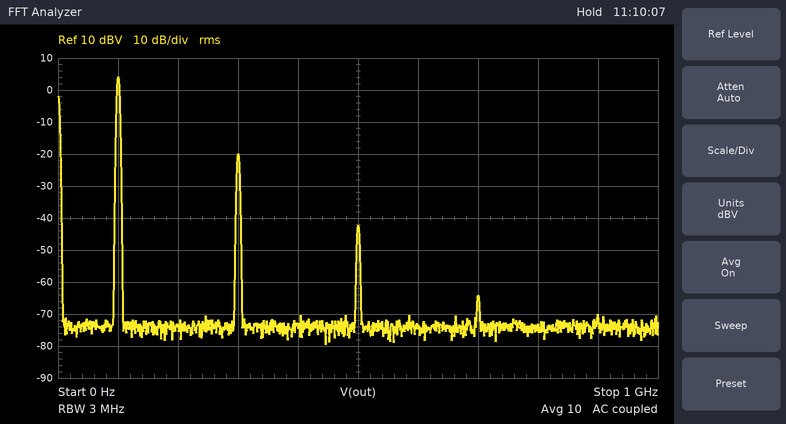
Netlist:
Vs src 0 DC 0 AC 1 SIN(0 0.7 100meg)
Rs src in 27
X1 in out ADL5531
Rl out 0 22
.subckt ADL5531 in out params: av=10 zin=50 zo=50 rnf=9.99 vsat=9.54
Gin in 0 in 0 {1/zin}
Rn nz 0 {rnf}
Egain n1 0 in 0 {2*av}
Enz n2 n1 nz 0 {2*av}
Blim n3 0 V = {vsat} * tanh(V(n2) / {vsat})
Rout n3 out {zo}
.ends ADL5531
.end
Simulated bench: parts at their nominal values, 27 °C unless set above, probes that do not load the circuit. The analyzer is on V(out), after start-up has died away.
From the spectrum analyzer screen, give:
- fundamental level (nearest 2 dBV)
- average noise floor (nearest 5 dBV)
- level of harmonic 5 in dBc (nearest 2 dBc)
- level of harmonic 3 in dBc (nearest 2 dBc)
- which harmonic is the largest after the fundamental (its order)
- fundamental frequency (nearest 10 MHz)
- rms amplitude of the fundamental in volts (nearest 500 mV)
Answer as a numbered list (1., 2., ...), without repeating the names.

1. 4 dBV
2. -75 dBV
3. -46 dBc
4. -24 dBc
5. 3
6. 100 MHz
7. 1.5 V
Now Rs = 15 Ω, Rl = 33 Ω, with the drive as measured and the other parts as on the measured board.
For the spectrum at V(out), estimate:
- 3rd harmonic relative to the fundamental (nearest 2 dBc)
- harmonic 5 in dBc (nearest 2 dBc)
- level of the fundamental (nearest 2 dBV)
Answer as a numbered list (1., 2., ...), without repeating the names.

1. -22 dBc
2. -42 dBc
3. 8 dBV
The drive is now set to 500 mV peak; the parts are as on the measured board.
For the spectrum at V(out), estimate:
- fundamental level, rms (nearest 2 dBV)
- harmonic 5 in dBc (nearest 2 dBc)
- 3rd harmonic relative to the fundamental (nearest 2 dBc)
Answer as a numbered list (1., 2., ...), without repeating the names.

1. 2 dBV
2. -56 dBc
3. -30 dBc
